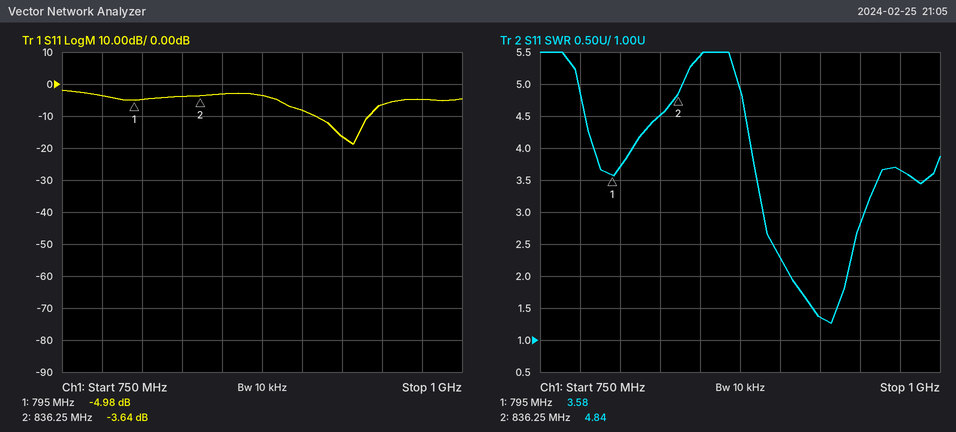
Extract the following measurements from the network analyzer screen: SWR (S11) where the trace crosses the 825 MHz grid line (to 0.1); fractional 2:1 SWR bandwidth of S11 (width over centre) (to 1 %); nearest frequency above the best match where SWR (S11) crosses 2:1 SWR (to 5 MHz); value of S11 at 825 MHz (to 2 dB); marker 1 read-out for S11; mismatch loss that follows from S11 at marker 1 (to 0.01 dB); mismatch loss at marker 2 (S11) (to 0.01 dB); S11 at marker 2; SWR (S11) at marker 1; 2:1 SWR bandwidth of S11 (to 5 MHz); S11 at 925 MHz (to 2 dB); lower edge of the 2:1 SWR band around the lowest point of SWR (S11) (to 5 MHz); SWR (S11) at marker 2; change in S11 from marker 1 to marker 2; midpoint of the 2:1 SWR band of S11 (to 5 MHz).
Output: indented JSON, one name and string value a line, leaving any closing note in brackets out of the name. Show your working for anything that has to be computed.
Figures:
{
  "SWR (S11) where the trace crosses the 825 MHz grid line": "4.5",
  "fractional 2:1 SWR bandwidth of S11 (width over centre)": "35 MHz / 922.5 MHz ≈ 4 %",
  "nearest frequency above the best match where SWR (S11) crosses 2:1 SWR": "940 MHz",
  "value of S11 at 825 MHz": "-4 dB",
  "marker 1 read-out for S11": "-4.98 dB",
  "mismatch loss that follows from S11 at marker 1": "−10 log10(1 − 10^(-4.98/10)) ≈ 1.66 dB",
  "mismatch loss at marker 2 (S11)": "−10 log10(1 − 10^(-3.64/10)) ≈ 2.46 dB",
  "S11 at marker 2": "-3.64 dB",
  "SWR (S11) at marker 1": "3.58",
  "2:1 SWR bandwidth of S11": "940 MHz − 905 MHz = 35 MHz",
  "S11 at 925 MHz": "-16 dB",
  "lower edge of the 2:1 SWR band around the lowest point of SWR (S11)": "905 MHz",
  "SWR (S11) at marker 2": "4.84",
  "change in S11 from marker 1 to marker 2": "-3.64 − (-4.98) = 1.34 dB",
  "midpoint of the 2:1 SWR band of S11": "925 MHz"
}
